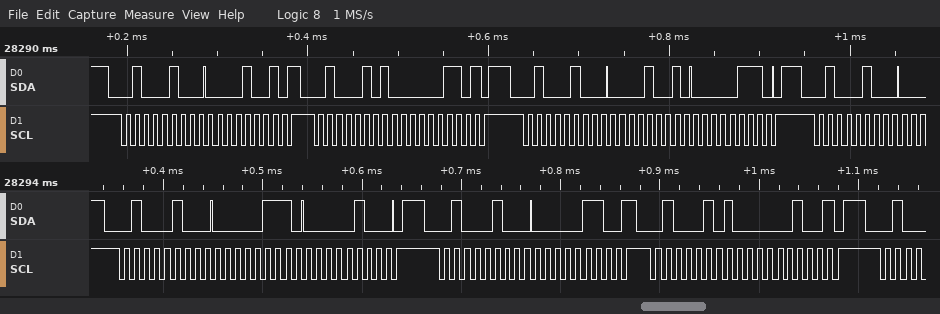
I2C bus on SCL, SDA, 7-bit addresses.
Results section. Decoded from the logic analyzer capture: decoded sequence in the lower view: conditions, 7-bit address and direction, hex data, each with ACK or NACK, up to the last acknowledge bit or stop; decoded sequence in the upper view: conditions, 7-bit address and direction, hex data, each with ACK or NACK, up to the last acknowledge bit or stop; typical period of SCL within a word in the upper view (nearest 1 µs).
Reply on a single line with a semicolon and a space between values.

start, address 22 write ACK, 07 ACK, 04 ACK, stop, start, address 22 write ACK, 06 ACK, repeated start, address 22 read ACK, 04 NACK, stop; start, address 22 write ACK, 09 ACK, repeated start, address 22 read ACK, 06 NACK, stop, start, address 22 write ACK, 09 ACK, 07 ACK, stop, start, address 22 write ACK; 10 µs
